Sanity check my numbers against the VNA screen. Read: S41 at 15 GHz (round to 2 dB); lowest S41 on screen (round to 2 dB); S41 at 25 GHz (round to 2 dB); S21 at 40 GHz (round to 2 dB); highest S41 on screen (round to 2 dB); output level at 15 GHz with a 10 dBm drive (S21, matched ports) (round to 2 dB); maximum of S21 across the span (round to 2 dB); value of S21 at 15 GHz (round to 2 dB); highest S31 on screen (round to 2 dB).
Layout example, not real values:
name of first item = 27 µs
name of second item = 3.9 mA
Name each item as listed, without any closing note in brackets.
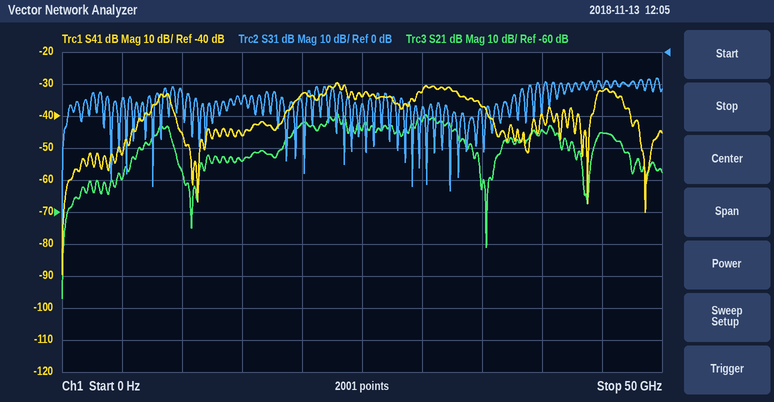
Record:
S41 at 15 GHz = -46 dB
lowest S41 on screen = -90 dB
S41 at 25 GHz = -34 dB
S21 at 40 GHz = -34 dB
highest S41 on screen = -30 dB
output level at 15 GHz with a 10 dBm drive (S21, matched ports) = -34 dBm
maximum of S21 across the span = -30 dB
value of S21 at 15 GHz = -44 dB
highest S31 on screen = -8 dB
